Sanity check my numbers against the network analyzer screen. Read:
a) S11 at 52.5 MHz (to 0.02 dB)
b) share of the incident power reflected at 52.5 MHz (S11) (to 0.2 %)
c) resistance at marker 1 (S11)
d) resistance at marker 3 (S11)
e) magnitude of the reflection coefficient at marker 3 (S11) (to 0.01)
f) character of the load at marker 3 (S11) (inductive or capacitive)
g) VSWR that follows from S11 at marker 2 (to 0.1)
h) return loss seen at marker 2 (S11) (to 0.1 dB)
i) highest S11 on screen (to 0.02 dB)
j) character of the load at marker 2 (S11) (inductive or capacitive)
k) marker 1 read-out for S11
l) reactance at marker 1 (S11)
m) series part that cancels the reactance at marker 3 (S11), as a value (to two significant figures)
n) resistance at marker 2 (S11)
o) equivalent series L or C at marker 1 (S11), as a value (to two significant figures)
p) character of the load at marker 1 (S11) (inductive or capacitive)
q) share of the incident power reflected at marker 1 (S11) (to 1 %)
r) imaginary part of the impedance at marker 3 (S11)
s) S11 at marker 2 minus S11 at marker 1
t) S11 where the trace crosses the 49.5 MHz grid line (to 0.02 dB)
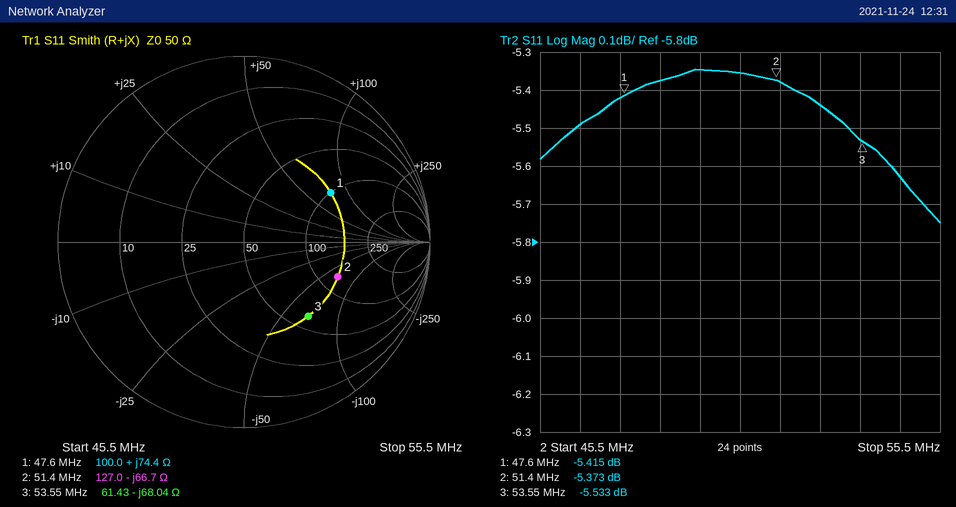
-5.44 dB
28.6 %
100.0 Ω
61.43 Ω
0.53
capacitive
3.3
5.4 dB
-5.34 dB
capacitive
-5.415 dB
+74.4 Ω
200 nH
127.0 Ω
250 nH
inductive
29 %
-68.04 Ω
0.042 dB
-5.34 dB
